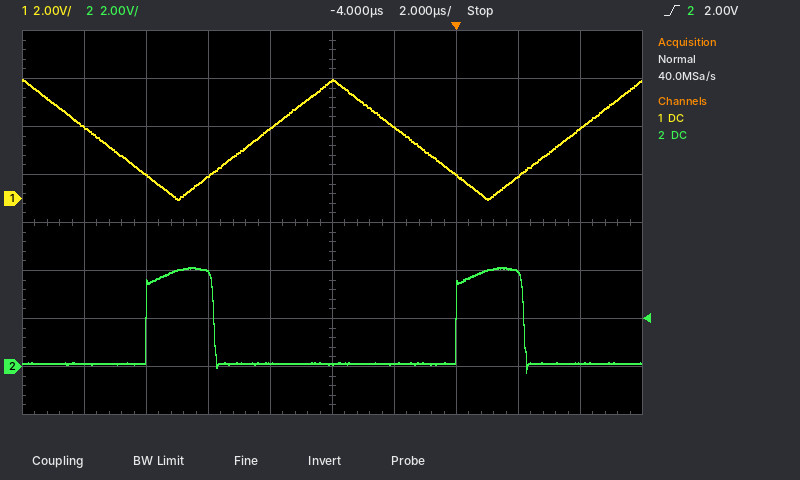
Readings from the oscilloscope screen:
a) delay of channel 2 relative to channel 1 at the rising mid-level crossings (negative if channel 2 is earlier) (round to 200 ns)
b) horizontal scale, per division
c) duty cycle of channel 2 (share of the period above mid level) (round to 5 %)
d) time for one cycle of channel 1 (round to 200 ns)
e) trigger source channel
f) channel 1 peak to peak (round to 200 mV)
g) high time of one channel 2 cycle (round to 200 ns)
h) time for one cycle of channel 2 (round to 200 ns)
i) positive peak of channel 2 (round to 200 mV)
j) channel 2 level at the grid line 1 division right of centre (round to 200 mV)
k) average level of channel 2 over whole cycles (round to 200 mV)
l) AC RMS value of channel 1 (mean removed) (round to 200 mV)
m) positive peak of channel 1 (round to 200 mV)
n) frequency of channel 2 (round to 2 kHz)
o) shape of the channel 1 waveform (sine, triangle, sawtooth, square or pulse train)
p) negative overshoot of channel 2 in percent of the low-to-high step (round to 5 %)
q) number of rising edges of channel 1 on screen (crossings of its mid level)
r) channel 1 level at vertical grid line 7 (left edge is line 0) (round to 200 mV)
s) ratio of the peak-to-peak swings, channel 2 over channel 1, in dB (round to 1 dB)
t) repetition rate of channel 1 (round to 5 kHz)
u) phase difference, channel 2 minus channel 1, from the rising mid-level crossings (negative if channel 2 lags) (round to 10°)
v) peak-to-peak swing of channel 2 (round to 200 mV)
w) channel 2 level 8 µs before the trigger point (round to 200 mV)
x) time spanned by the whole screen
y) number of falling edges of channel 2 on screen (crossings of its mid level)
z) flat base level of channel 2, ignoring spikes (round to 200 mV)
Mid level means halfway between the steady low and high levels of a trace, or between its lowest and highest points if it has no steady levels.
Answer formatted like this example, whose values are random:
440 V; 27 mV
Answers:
-3.6 µs; 2 µs; 20 %; 10.0 µs; channel 2; 5.0 V; 2.2 µs; 10.0 µs; 4.2 V; 200 mV; 1.0 V; 1.4 V; 5.0 V; 100 kHz; triangle; 10 %; 2; 1.0 V; -1 dB; 100 kHz; +130°; 4.4 V; 3.8 V; 20 µs; 2; 200 mV
